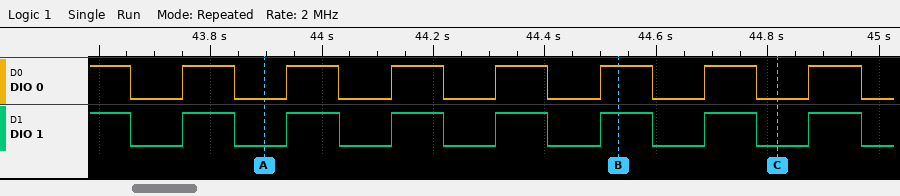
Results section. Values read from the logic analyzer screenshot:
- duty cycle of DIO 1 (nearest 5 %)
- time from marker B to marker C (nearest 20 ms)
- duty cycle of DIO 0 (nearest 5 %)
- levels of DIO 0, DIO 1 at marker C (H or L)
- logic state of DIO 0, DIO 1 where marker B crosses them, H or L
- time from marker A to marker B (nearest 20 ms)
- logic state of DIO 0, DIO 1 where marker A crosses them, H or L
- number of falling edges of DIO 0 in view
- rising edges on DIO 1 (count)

50 %
280 ms
50 %
DIO 0=L, DIO 1=L
DIO 0=H, DIO 1=H
640 ms
DIO 0=L, DIO 1=L
8
7
